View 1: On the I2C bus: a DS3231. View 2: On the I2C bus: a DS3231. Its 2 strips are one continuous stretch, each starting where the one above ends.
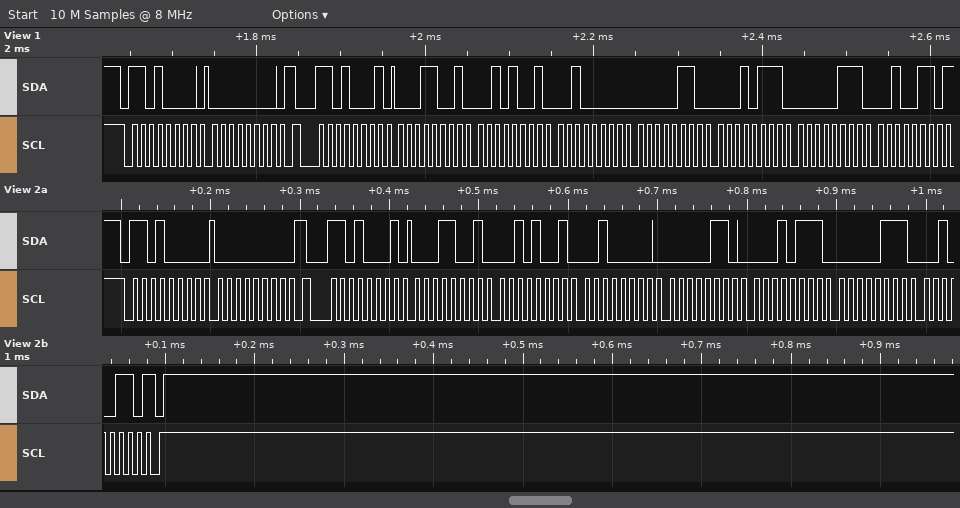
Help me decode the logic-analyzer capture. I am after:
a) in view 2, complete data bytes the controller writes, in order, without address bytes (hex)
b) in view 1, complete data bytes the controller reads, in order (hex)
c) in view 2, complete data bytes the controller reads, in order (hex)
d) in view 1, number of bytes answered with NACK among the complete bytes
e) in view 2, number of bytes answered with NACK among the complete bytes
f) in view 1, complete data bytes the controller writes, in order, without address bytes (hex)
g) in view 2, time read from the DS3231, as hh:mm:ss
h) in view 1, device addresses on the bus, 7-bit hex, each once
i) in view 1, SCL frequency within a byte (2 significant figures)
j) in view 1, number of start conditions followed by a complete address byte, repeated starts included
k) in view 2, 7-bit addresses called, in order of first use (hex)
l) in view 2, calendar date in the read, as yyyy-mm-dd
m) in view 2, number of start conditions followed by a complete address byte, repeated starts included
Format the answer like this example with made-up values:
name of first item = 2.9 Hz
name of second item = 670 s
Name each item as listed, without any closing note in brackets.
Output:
in view 2, complete data bytes the controller writes, in order, without address bytes = 00
in view 1, complete data bytes the controller reads, in order = 19 29 20 06 17 07 26
in view 2, complete data bytes the controller reads, in order = 19 29 20 06 17 07 26
in view 1, number of bytes answered with NACK among the complete bytes = 1
in view 2, number of bytes answered with NACK among the complete bytes = 1
in view 1, complete data bytes the controller writes, in order, without address bytes = 00
in view 2, time read from the DS3231, as hh:mm:ss = 20:29:19
in view 1, device addresses on the bus, 7-bit hex, each once = 0x68
in view 1, SCL frequency within a byte = 100 kHz
in view 1, number of start conditions followed by a complete address byte, repeated starts included = 2
in view 2, 7-bit addresses called, in order of first use = 0x68
in view 2, calendar date in the read, as yyyy-mm-dd = 2026-07-17
in view 2, number of start conditions followed by a complete address byte, repeated starts included = 2
